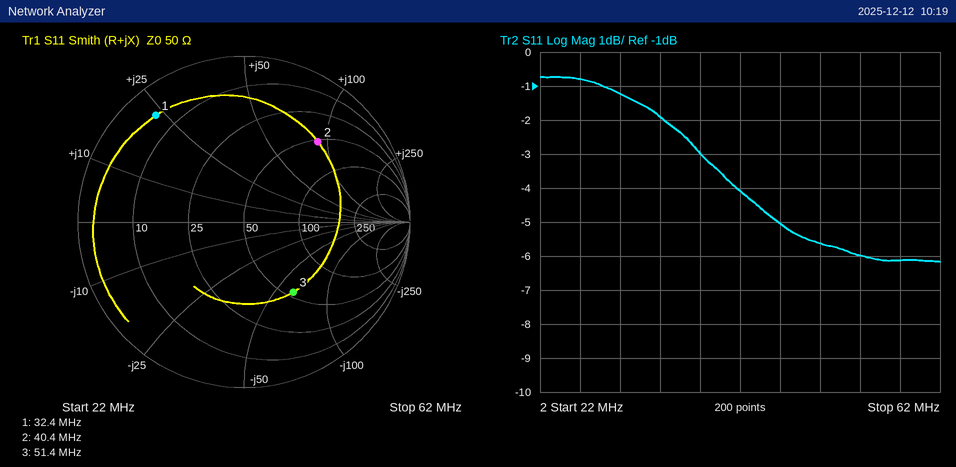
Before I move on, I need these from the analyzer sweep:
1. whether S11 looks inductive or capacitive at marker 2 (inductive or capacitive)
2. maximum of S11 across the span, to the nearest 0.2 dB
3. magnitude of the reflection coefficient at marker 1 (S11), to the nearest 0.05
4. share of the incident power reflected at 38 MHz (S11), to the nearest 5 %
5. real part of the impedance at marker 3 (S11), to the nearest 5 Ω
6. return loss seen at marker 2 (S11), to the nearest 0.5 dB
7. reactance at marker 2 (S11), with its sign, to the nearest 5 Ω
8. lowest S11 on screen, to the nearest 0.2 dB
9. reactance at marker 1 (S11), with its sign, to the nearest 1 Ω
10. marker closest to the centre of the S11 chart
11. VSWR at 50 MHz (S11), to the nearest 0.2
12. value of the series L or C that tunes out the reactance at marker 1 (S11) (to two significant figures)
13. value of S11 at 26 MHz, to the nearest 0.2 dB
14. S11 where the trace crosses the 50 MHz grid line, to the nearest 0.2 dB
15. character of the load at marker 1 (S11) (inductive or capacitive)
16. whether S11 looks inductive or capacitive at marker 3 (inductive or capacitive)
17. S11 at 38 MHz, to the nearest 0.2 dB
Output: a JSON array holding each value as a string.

["inductive", "-0.8 dB", "0.85", "50 %", "55 Ω", "3.5 dB", "+90 Ω", "-6.2 dB", "+23 Ω", "marker 3", "3.2", "210 pF", "-0.8 dB", "-5.6 dB", "inductive", "capacitive", "-3.0 dB"]
